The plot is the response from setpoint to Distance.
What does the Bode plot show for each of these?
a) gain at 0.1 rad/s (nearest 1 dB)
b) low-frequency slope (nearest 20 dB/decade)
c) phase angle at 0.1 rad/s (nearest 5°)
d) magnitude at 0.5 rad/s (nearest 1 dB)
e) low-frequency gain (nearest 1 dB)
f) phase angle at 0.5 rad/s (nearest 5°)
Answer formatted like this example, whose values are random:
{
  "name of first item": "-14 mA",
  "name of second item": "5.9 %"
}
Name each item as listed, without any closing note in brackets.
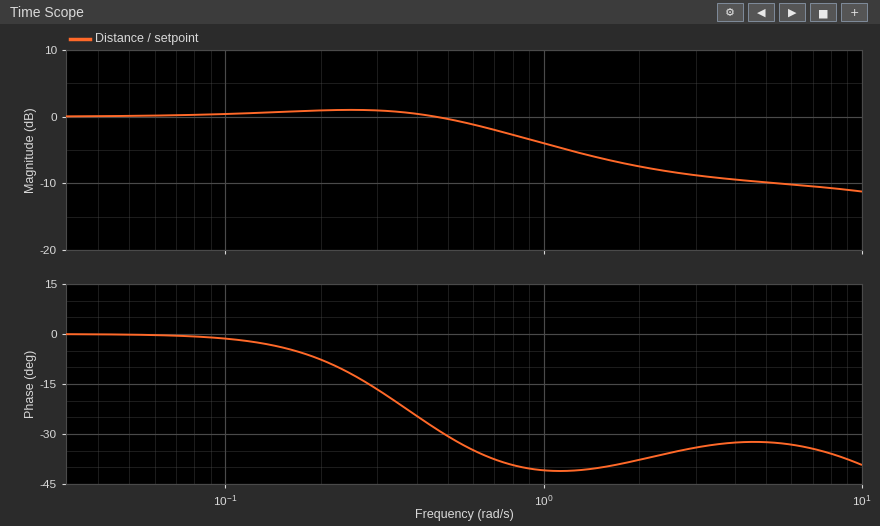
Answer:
{
  "gain at 0.1 rad/s": "0 dB",
  "low-frequency slope": "0 dB/decade",
  "phase angle at 0.1 rad/s": "0°",
  "magnitude at 0.5 rad/s": "0 dB",
  "low-frequency gain": "0 dB",
  "phase angle at 0.5 rad/s": "-30°"
}
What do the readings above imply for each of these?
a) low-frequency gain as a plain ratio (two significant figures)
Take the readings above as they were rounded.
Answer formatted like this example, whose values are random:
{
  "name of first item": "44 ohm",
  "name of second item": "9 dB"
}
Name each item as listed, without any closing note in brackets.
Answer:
{
  "low-frequency gain as a plain ratio": "1.0"
}
